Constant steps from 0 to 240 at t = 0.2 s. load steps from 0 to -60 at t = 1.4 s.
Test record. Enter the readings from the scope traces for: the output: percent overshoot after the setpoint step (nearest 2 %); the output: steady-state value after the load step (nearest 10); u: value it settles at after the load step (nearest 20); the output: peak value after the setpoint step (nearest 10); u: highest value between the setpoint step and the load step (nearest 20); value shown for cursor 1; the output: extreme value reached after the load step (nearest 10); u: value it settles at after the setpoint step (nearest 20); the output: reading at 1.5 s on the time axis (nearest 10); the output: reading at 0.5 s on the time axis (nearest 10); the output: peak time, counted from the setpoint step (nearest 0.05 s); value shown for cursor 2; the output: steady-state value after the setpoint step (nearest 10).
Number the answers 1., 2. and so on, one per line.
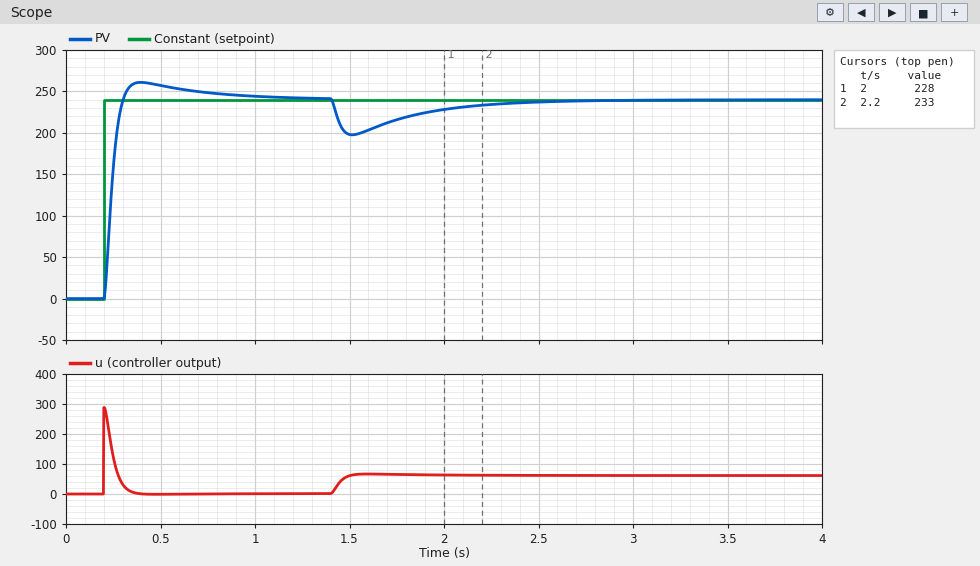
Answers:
1. 8 %
2. 240
3. 60
4. 260
5. 280
6. 228
7. 200
8. 0
9. 200
10. 260
11. 0.20 s
12. 233
13. 240
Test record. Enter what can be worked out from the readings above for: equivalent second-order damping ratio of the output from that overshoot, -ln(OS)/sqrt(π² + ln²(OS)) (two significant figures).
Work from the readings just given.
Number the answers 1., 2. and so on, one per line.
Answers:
1. 0.63
